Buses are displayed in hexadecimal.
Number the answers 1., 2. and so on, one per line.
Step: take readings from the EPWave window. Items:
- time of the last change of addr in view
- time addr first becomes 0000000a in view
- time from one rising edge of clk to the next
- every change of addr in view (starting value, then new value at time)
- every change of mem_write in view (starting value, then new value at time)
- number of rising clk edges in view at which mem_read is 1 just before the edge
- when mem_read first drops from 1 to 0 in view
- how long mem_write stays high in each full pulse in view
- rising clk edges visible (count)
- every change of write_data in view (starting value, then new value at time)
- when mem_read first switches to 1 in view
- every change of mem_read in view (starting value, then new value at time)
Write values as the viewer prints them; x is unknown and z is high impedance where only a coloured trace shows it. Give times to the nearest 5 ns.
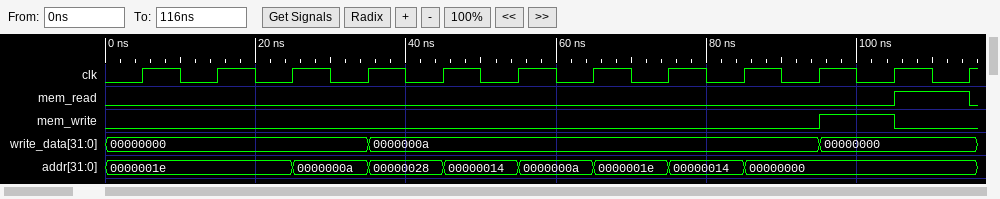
1. 85 ns
2. 25 ns
3. 10 ns
4. 0000001e, 0000000a at 25 ns, 00000028 at 35 ns, 00000014 at 45 ns, 0000000a at 55 ns, 0000001e at 65 ns, 00000014 at 75 ns, 00000000 at 85 ns
5. 0, 1 at 95 ns, 0 at 105 ns
6. 1
7. 115 ns
8. 10 ns
9. 12
10. 00000000, 0000000a at 35 ns, 00000000 at 95 ns
11. 105 ns
12. 0, 1 at 105 ns, 0 at 115 ns
